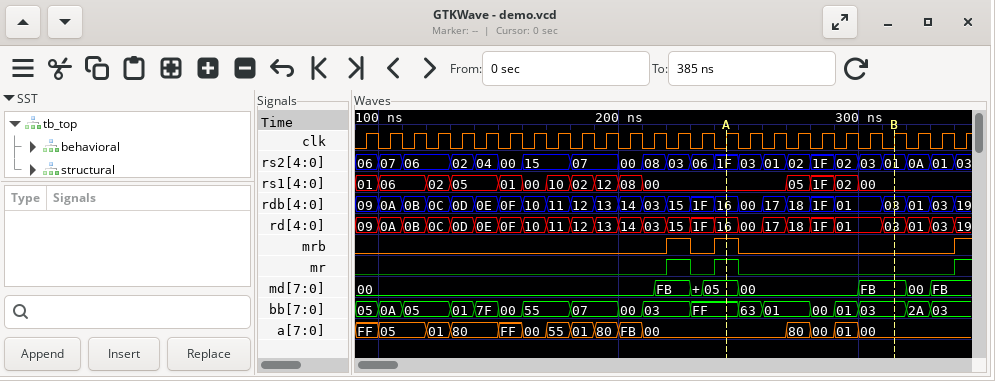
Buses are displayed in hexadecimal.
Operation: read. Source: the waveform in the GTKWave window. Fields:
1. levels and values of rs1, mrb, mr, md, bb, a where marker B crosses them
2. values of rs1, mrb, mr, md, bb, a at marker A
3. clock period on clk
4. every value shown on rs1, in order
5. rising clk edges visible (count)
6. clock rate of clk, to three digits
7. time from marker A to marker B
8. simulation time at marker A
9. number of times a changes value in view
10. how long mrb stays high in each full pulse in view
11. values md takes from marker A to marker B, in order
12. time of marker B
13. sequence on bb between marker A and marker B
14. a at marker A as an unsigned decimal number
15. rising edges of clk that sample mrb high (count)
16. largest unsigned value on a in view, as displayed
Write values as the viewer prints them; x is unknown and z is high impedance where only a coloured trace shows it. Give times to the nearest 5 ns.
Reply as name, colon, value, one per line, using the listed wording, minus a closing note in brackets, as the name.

levels and values of rs1, mrb, mr, md, bb, a where marker B crosses them: rs1=00, mrb=0, mr=0, md=FB, bb=03, a=00
values of rs1, mrb, mr, md, bb, a at marker A: rs1=00, mrb=1, mr=1, md=05, bb=FF, a=00
clock period on clk: 10 ns
every value shown on rs1, in order: 01, 06, 02, 05, 01, 00, 10, 02, 12, 08, 00, 05, 1F, 02, 00
rising clk edges visible: 26
clock rate of clk, to three digits: 100 MHz
time from marker A to marker B: 70 ns
simulation time at marker A: 245 ns
number of times a changes value in view: 14
how long mrb stays high in each full pulse in view: 10 ns, 10 ns
values md takes from marker A to marker B, in order: 05, 00, FB
time of marker B: 315 ns
sequence on bb between marker A and marker B: FF, 63, 01, 00, 01, 03
a at marker A as an unsigned decimal number: 0
rising edges of clk that sample mrb high: 3
largest unsigned value on a in view, as displayed: FF
